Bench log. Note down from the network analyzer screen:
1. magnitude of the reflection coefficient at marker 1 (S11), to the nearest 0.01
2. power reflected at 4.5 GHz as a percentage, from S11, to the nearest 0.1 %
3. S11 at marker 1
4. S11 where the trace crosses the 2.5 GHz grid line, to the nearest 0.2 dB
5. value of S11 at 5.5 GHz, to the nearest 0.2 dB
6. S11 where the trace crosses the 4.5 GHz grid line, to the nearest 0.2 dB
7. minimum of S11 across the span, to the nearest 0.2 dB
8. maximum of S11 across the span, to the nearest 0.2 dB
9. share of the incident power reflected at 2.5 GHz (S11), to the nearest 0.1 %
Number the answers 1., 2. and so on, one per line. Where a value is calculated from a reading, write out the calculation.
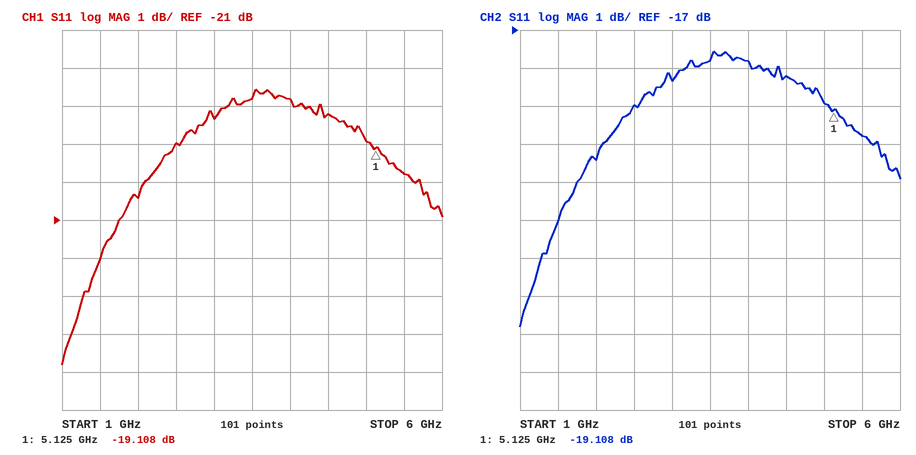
1. 10^(-19.108/20) ≈ 0.11
2. 10^(-18.2/10) ≈ 1.5 %
3. -19.108 dB
4. -19.0 dB
5. -19.8 dB
6. -18.2 dB
7. -24.8 dB
8. -17.6 dB
9. 10^(-19/10) ≈ 1.3 %
